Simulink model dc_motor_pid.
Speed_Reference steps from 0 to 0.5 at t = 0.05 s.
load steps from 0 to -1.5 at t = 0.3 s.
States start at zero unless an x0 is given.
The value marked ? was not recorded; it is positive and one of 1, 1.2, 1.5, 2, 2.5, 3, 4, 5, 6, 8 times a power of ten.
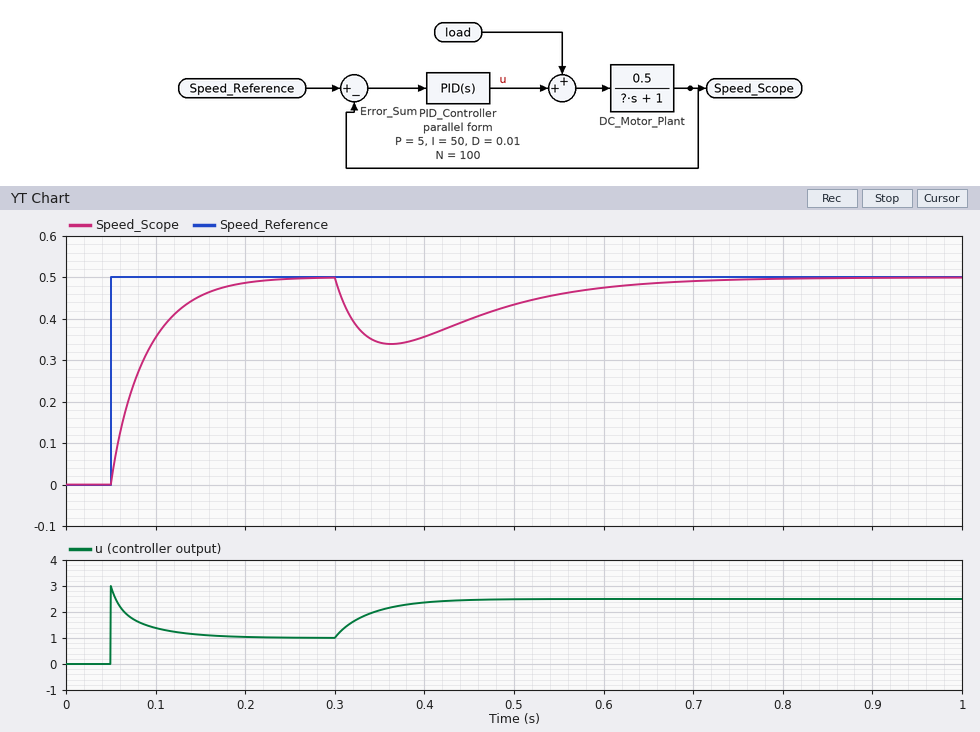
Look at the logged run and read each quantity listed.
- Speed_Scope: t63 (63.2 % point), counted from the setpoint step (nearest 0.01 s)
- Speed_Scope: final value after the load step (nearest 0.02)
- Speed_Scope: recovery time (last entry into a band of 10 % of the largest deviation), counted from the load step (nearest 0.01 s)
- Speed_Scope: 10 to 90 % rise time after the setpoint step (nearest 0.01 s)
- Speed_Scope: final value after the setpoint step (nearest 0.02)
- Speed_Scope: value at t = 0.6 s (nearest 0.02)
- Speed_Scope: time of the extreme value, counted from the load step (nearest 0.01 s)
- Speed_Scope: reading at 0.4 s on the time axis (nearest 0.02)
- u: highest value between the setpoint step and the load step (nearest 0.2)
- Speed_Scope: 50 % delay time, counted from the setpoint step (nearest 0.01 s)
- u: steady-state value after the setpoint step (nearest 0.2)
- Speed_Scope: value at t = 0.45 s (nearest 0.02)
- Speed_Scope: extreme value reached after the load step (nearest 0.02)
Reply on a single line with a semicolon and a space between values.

0.04 s; 0.50; 0.34 s; 0.09 s; 0.50; 0.48; 0.06 s; 0.36; 3.0; 0.03 s; 1.0; 0.40; 0.34
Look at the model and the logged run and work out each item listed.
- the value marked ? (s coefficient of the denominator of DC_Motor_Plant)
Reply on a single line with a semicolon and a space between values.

0.1
